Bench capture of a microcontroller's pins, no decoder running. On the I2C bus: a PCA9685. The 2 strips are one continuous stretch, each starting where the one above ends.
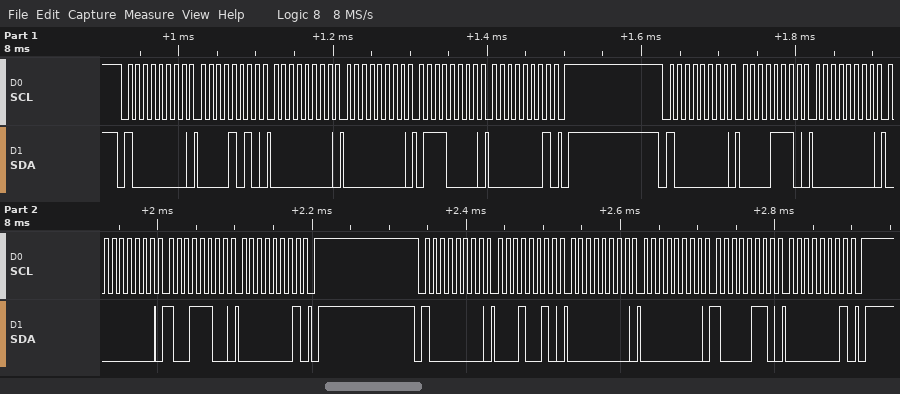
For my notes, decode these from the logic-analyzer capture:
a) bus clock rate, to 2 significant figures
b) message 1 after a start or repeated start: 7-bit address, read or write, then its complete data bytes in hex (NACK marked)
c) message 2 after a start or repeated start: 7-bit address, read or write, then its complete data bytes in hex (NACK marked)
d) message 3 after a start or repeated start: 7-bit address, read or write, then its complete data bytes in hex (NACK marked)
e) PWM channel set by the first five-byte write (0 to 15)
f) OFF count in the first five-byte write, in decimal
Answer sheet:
100 kHz
0x40 write: 0A 00 00 70 01
0x40 write: 0E 00 00 9C 01
0x40 write: 12 00 00 86 01
1
368
